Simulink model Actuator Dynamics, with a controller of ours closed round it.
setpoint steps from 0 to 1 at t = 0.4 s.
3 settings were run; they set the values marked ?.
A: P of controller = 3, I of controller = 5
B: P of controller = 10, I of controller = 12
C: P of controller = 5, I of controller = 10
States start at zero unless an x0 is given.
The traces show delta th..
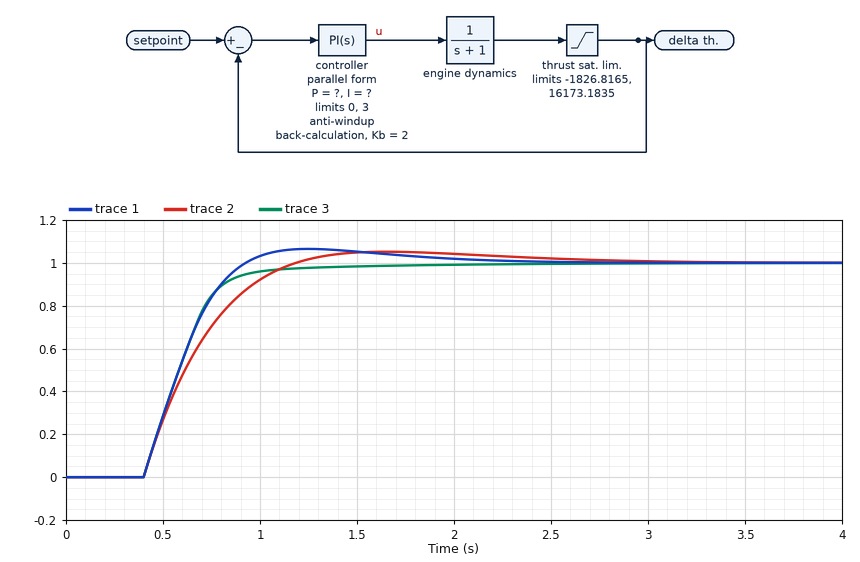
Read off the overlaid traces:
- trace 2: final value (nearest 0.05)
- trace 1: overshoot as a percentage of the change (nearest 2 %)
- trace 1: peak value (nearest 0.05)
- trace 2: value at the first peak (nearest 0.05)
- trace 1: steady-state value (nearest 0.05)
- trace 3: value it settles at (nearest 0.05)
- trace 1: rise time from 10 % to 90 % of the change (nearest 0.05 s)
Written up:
1.00
6 %
1.05
1.05
1.00
1.00
0.35 s
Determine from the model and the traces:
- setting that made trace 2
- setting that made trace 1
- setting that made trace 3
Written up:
A
C
B
